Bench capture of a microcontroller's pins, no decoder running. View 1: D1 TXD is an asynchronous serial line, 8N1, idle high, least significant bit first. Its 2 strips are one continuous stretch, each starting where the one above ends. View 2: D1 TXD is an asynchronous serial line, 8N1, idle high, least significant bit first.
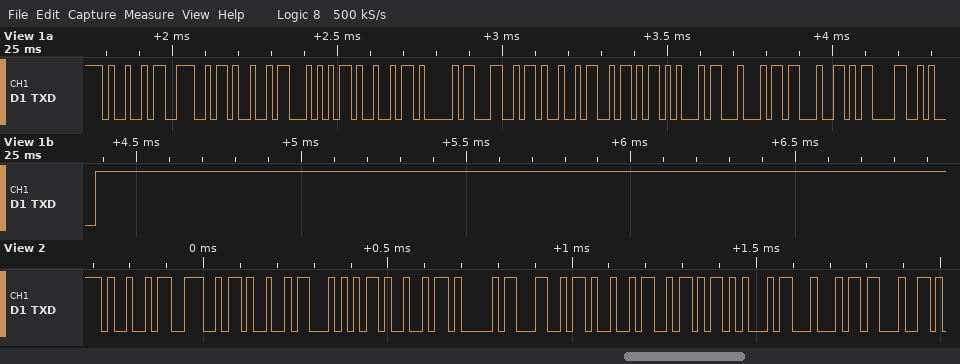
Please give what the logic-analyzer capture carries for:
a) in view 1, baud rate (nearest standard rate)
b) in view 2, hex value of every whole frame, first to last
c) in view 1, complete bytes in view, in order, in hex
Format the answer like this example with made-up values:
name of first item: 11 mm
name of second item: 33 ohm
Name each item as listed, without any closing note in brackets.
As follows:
in view 1, baud rate: 57600 baud
in view 2, hex value of every whole frame, first to last: 49 4E 49 54 49 41 4C 49 5A 45 44 23
in view 1, complete bytes in view, in order, in hex: 49 4E 49 54 49 41 4C 49 5A 45 44 23 0D 0A
